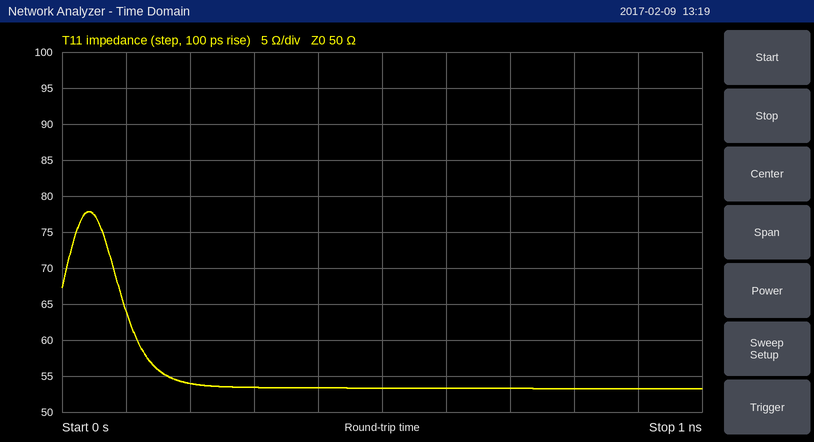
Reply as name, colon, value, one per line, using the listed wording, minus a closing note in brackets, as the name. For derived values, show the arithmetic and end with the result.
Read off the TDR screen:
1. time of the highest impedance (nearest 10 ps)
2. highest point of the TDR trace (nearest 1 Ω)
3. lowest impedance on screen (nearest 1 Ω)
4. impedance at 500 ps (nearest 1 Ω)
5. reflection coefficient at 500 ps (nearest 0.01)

time of the highest impedance: 40 ps
highest point of the TDR trace: 78 Ω
lowest impedance on screen: 53 Ω
impedance at 500 ps: 53 Ω
reflection coefficient at 500 ps: (53 − 50)/(53 + 50) ≈ +0.03
